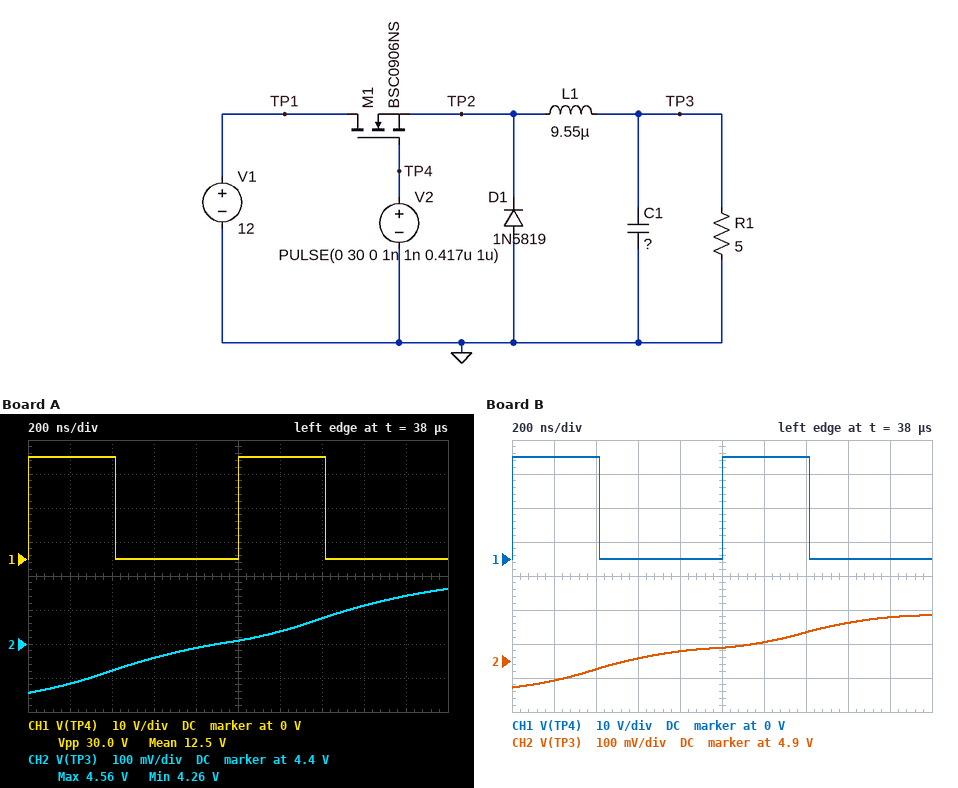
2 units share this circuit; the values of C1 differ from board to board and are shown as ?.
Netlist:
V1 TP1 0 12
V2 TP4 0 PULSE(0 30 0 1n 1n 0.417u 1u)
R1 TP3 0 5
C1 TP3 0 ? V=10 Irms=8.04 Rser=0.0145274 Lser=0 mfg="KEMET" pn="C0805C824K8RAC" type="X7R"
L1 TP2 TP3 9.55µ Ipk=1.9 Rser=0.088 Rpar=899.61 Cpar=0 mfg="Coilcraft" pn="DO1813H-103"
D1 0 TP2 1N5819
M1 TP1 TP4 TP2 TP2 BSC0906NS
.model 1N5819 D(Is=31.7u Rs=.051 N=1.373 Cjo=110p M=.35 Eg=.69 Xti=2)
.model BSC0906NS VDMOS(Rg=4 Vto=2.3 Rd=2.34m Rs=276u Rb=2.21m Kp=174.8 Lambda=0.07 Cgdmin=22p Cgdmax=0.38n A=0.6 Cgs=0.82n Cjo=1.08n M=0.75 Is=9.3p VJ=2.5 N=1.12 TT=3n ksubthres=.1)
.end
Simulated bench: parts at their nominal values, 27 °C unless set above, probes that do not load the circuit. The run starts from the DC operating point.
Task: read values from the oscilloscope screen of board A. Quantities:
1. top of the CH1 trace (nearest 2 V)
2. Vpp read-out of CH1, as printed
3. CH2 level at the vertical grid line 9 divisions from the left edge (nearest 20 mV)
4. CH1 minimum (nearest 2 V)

30 V
30.0 V
4.54 V
0 V
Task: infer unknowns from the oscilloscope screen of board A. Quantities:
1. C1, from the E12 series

2.7 µF
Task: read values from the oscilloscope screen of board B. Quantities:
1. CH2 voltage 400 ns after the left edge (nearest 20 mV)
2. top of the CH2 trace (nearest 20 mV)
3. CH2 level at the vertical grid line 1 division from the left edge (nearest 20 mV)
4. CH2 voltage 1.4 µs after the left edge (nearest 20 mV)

4.88 V
5.04 V
4.84 V
4.98 V
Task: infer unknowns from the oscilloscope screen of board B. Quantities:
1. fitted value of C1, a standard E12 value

2.2 µF
